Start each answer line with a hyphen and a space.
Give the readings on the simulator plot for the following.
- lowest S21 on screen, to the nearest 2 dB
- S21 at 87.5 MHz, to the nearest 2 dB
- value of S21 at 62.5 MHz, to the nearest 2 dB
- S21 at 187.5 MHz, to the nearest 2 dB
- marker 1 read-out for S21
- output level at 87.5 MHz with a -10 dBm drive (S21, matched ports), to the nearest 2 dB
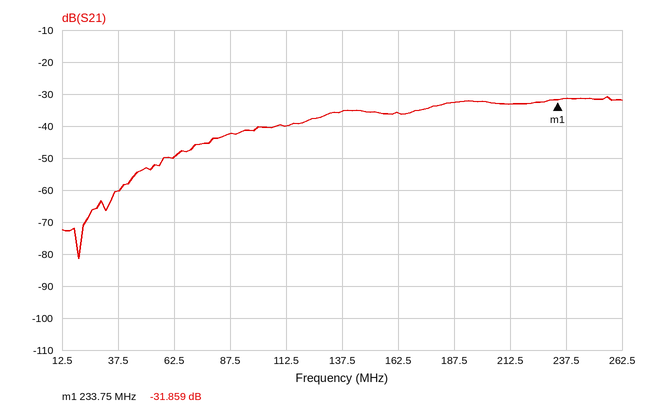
- -82 dB
- -42 dB
- -50 dB
- -32 dB
- -31.859 dB
- -52 dBm
